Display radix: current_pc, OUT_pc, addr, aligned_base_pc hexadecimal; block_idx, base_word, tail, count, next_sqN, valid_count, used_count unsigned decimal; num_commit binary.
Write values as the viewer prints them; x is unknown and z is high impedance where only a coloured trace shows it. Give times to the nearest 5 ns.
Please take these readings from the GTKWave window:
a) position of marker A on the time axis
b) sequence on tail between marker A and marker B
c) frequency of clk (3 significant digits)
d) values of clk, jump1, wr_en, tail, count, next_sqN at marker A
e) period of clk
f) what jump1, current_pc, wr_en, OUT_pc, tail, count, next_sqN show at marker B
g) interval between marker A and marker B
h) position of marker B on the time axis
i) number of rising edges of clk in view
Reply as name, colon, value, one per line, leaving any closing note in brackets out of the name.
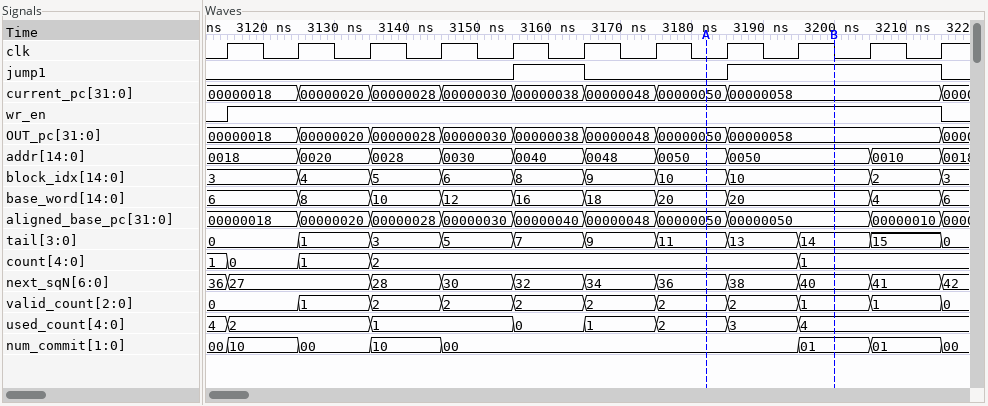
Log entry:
position of marker A on the time axis: 3180 ns
sequence on tail between marker A and marker B: 11, 13, 14
frequency of clk: 100 MHz
values of clk, jump1, wr_en, tail, count, next_sqN at marker A: clk=0, jump1=0, wr_en=1, tail=11, count=2, next_sqN=36
period of clk: 10 ns
what jump1, current_pc, wr_en, OUT_pc, tail, count, next_sqN show at marker B: jump1=1, current_pc=00000058, wr_en=1, OUT_pc=00000058, tail=14, count=1, next_sqN=40
interval between marker A and marker B: 20 ns
position of marker B on the time axis: 3200 ns
number of rising edges of clk in view: 11
